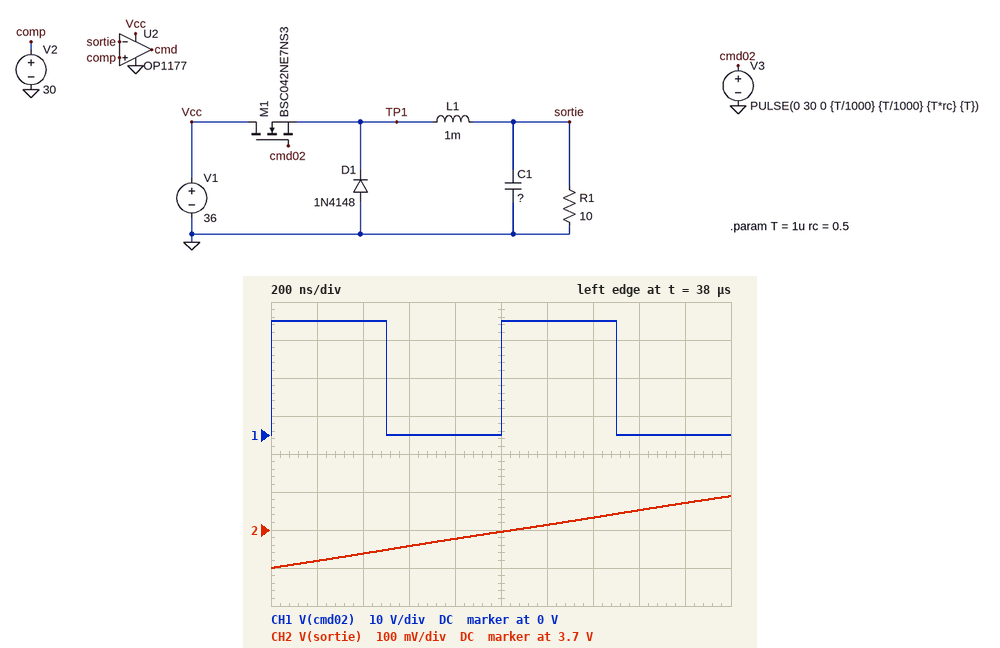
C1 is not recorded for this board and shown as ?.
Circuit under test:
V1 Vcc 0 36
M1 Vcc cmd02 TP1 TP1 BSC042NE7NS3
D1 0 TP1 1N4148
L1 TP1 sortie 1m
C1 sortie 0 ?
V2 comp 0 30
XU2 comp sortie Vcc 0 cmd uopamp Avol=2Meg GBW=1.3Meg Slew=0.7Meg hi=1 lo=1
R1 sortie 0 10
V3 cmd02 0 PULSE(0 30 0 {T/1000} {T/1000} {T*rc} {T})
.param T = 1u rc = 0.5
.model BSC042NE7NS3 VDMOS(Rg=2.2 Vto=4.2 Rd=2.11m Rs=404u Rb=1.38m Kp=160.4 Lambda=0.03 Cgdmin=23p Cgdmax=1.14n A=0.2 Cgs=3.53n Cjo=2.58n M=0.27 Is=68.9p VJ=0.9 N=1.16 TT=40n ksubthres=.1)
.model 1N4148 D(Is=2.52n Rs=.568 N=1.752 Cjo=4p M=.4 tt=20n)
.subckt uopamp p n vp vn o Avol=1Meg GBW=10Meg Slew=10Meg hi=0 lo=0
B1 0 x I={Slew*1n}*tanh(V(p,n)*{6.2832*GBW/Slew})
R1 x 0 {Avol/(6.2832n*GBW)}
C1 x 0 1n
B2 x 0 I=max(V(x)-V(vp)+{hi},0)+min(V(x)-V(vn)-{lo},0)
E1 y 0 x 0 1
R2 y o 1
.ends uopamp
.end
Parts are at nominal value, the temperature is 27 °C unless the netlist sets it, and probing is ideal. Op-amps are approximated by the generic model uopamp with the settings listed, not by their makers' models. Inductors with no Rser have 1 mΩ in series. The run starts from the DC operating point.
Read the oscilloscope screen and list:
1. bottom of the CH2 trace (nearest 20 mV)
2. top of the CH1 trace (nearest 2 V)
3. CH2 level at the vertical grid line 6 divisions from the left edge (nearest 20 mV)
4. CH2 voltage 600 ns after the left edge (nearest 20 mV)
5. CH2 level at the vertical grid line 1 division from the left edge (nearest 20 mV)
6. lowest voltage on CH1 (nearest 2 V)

3.60 V
30 V
3.72 V
3.66 V
3.62 V
0 V
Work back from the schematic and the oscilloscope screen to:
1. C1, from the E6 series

680 nF
